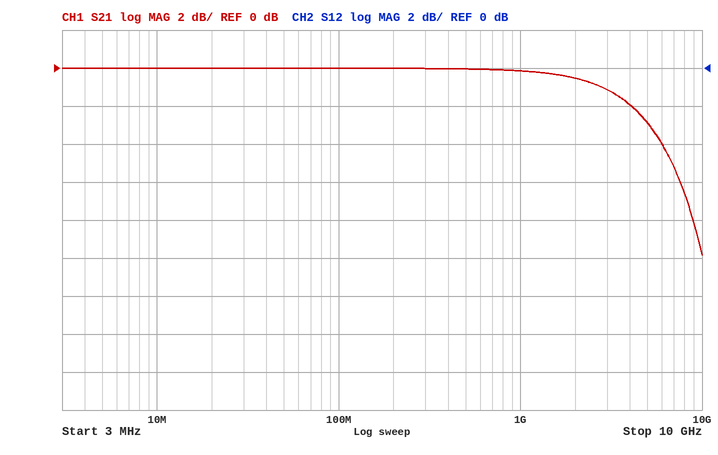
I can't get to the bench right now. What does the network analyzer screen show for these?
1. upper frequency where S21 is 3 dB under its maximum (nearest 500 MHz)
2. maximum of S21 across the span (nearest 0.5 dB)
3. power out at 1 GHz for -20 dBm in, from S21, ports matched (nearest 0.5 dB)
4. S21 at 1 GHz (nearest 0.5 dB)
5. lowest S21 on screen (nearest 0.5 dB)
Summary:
5.0 GHz
0.0 dB
-20.0 dBm
0.0 dB
-10.0 dB
